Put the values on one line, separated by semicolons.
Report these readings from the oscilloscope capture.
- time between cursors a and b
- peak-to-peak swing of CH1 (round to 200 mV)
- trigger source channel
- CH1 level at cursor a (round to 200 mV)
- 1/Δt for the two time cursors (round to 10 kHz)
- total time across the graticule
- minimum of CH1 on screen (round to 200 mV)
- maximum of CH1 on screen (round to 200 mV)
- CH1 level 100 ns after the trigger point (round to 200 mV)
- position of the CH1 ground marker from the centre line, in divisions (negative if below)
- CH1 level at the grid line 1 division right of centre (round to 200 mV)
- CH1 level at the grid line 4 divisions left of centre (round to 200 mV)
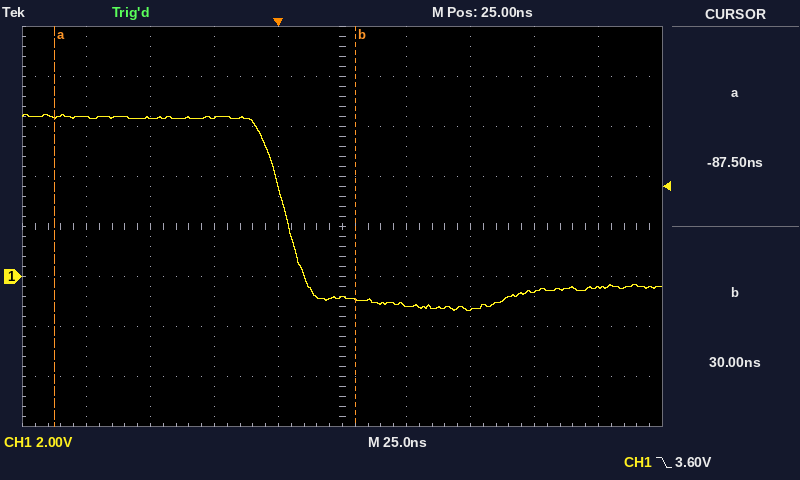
117.5 ns; 7.8 V; CH1; 6.4 V; 8.51 MHz; 250 ns; -1.4 V; 6.4 V; -600 mV; -1.0 div; -1.2 V; 6.4 V
